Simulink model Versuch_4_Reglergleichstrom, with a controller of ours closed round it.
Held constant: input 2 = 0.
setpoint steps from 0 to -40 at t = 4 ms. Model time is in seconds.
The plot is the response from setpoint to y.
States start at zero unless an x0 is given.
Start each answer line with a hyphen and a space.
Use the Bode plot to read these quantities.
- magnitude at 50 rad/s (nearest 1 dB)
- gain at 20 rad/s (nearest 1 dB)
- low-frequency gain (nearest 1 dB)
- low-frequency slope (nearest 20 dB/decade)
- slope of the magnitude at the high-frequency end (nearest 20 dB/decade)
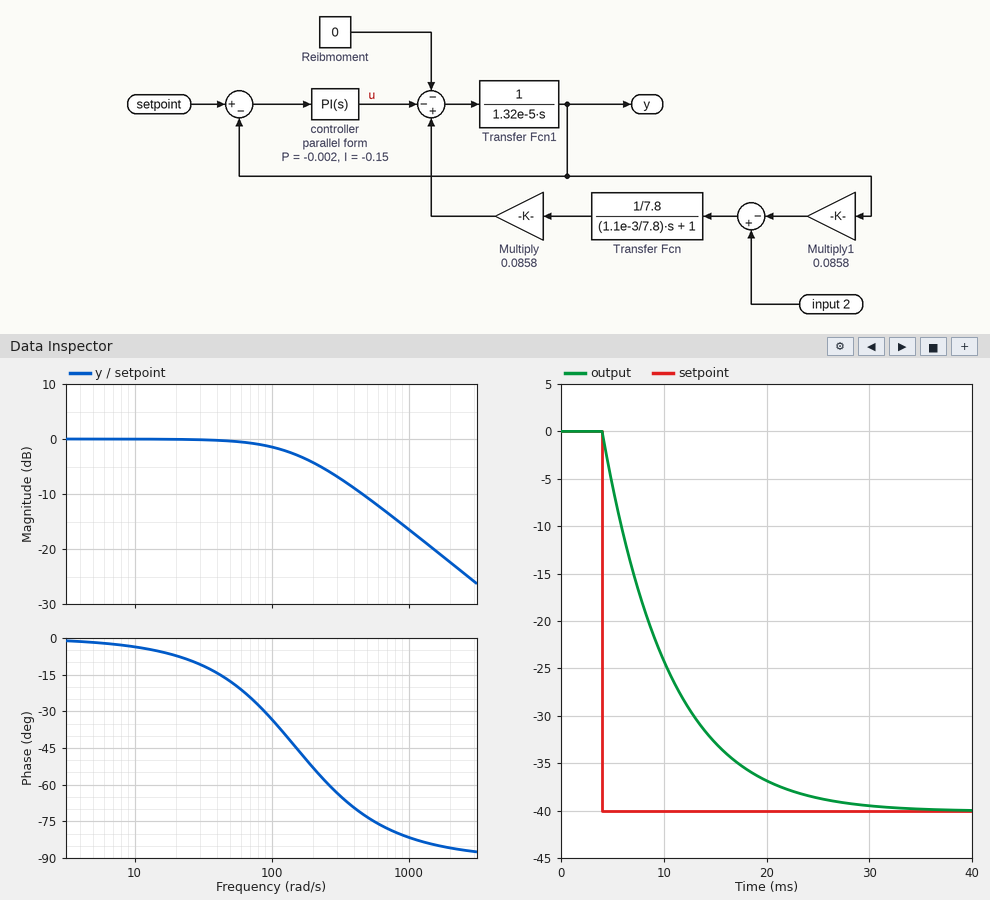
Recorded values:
- 0 dB
- 0 dB
- 0 dB
- 0 dB/decade
- -20 dB/decade
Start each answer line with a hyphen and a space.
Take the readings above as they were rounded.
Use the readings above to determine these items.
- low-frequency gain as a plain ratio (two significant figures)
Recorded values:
- 1.0
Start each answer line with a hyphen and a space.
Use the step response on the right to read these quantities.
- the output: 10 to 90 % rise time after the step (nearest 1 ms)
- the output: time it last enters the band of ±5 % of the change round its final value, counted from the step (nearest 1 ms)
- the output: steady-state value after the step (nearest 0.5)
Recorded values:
- 14 ms
- 19 ms
- -40.0
